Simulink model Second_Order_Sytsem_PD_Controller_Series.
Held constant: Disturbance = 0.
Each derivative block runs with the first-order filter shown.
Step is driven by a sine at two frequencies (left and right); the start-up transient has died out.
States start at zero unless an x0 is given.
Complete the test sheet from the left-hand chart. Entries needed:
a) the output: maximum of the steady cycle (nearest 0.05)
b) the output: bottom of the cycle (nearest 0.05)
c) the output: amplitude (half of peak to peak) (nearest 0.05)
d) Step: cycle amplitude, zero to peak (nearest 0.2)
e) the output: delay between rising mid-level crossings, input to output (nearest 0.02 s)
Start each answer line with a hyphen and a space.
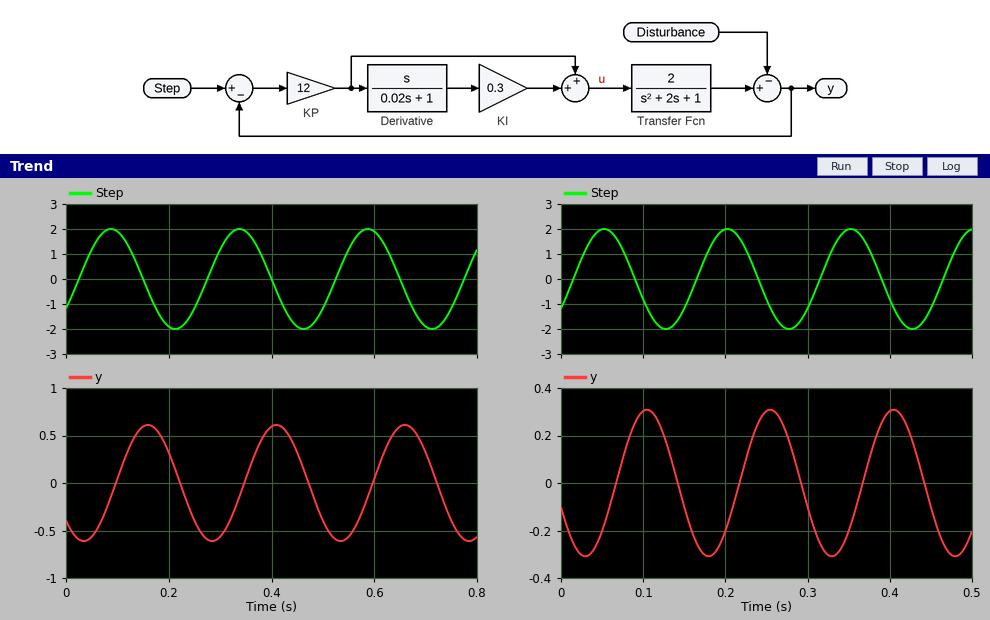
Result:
- 0.60
- -0.60
- 0.60
- 2.0
- 0.08 s
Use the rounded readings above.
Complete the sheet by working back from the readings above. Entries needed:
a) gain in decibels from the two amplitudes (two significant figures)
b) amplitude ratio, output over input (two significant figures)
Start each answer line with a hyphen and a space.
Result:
- -10 dB
- 0.30
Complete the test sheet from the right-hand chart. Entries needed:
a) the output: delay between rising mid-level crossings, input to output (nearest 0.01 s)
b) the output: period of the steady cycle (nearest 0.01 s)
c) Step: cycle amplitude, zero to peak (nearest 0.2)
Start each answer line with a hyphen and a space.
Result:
- 0.05 s
- 0.15 s
- 2.0
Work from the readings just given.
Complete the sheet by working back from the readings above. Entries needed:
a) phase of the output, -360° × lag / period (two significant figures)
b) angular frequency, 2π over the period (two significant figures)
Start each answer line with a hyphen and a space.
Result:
- -120°
- 42 rad/s
